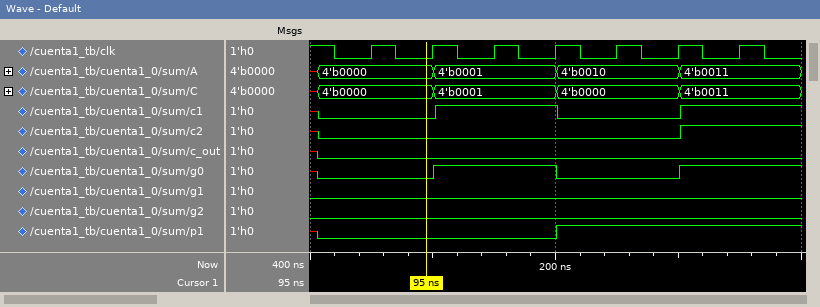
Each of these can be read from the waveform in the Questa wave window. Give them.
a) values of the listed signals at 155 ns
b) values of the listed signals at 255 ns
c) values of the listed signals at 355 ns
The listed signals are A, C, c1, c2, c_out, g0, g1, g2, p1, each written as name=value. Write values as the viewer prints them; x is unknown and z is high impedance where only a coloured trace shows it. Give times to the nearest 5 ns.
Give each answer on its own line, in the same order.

A=4'b0001, C=4'b0001, c1=1, c2=0, c_out=0, g0=1, g1=0, g2=0, p1=0
A=4'b0010, C=4'b0000, c1=0, c2=0, c_out=0, g0=0, g1=0, g2=0, p1=1
A=4'b0011, C=4'b0011, c1=1, c2=1, c_out=0, g0=1, g1=0, g2=0, p1=1
